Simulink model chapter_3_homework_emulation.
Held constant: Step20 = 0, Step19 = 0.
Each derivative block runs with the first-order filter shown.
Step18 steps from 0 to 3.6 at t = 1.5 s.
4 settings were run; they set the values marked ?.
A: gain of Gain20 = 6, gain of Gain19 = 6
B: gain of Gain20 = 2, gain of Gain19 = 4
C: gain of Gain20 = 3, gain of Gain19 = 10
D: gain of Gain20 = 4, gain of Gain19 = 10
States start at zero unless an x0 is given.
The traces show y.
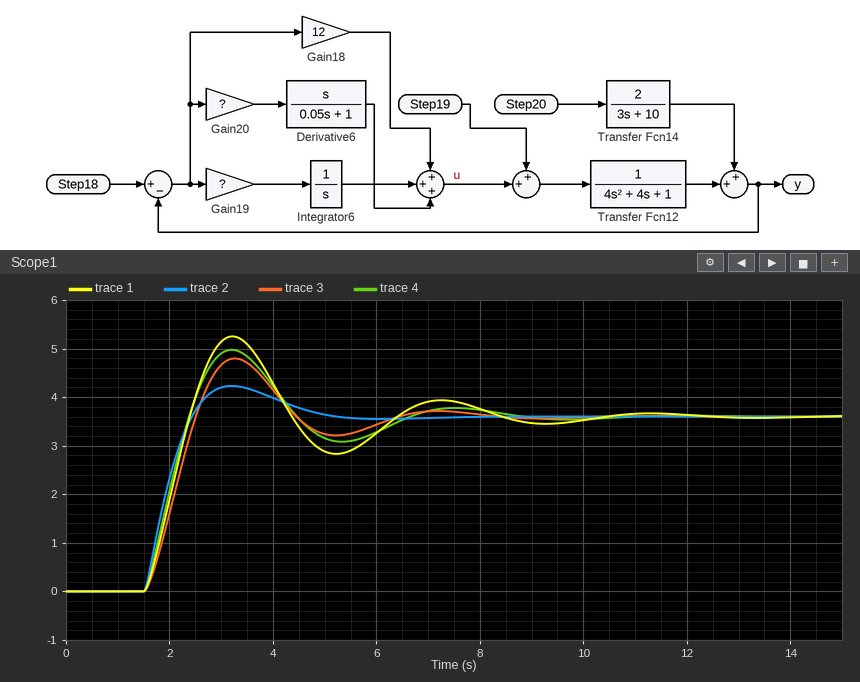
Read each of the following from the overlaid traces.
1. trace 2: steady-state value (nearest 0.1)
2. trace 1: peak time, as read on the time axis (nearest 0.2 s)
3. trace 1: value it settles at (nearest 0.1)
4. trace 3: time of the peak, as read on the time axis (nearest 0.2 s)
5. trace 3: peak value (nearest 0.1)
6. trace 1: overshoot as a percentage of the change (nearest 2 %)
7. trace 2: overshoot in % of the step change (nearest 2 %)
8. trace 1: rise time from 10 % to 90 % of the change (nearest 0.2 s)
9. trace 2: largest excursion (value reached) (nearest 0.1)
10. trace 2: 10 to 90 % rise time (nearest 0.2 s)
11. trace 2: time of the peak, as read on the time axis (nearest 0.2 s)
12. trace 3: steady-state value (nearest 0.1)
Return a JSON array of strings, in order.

["3.6", "3.2 s", "3.6", "3.2 s", "4.8", "46 %", "18 %", "0.6 s", "4.2", "0.6 s", "3.2 s", "3.6"]
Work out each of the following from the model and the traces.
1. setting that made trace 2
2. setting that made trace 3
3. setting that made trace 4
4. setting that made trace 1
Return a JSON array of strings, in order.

["A", "B", "D", "C"]
